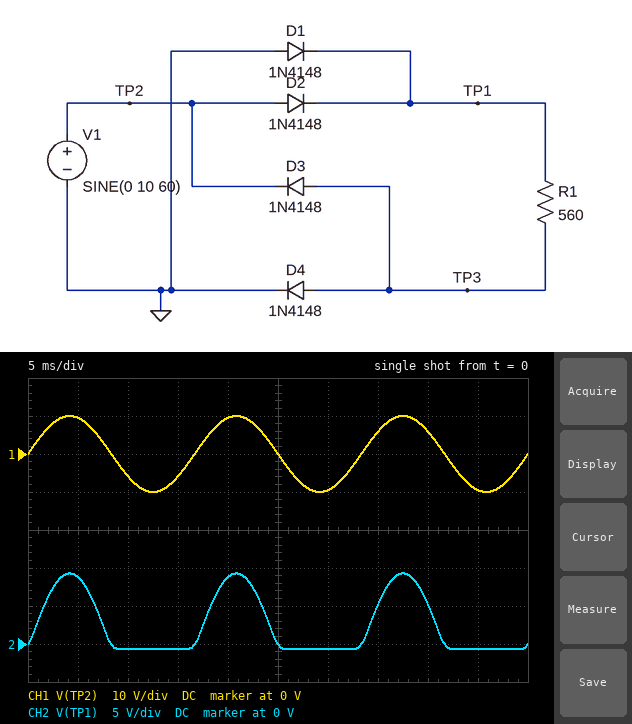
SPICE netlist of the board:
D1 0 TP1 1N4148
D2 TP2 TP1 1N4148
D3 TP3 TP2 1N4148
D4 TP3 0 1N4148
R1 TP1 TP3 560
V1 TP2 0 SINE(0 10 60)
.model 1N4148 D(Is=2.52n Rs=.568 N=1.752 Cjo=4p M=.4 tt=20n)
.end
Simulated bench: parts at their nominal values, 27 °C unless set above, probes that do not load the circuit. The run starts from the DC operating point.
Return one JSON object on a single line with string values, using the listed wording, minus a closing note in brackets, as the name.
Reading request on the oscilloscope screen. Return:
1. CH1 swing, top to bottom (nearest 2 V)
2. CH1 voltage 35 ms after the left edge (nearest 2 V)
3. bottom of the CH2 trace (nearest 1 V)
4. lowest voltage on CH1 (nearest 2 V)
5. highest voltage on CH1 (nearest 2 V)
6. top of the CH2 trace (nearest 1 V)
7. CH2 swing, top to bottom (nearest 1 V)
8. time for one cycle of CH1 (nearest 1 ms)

{"CH1 swing, top to bottom": "20 V", "CH1 voltage 35 ms after the left edge": "6 V", "bottom of the CH2 trace": "-1 V", "lowest voltage on CH1": "-10 V", "highest voltage on CH1": "10 V", "top of the CH2 trace": "9 V", "CH2 swing, top to bottom": "10 V", "time for one cycle of CH1": "17 ms"}
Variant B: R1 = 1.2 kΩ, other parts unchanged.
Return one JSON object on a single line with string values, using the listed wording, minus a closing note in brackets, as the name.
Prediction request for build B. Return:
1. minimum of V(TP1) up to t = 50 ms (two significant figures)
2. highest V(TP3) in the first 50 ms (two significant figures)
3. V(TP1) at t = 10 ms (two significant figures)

{"minimum of V(TP1) up to t = 50 ms": "-680 mV", "highest V(TP3) in the first 50 ms": "680 mV", "V(TP1) at t = 10 ms": "-650 mV"}
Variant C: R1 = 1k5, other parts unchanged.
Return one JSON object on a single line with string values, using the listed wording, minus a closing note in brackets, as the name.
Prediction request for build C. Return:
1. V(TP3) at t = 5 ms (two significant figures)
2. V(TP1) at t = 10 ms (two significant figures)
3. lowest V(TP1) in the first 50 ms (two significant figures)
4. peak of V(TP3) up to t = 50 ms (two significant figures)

{"V(TP3) at t = 5 ms": "660 mV", "V(TP1) at t = 10 ms": "-640 mV", "lowest V(TP1) in the first 50 ms": "-670 mV", "peak of V(TP3) up to t = 50 ms": "670 mV"}
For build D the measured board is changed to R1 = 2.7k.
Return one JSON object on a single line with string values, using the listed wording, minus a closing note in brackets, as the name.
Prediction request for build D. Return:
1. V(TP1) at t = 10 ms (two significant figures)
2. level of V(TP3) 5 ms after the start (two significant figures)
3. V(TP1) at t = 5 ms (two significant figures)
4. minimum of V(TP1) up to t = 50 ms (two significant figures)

{"V(TP1) at t = 10 ms": "-610 mV", "level of V(TP3) 5 ms after the start": "640 mV", "V(TP1) at t = 5 ms": "8.9 V", "minimum of V(TP1) up to t = 50 ms": "-640 mV"}
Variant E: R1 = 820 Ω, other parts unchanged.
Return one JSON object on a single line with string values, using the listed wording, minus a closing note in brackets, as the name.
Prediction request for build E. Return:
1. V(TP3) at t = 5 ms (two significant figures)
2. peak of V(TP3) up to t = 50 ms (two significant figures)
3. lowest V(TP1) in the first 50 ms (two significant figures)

{"V(TP3) at t = 5 ms": "690 mV", "peak of V(TP3) up to t = 50 ms": "700 mV", "lowest V(TP1) in the first 50 ms": "-700 mV"}
